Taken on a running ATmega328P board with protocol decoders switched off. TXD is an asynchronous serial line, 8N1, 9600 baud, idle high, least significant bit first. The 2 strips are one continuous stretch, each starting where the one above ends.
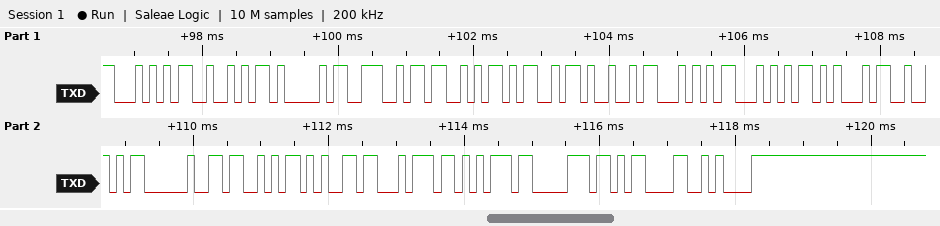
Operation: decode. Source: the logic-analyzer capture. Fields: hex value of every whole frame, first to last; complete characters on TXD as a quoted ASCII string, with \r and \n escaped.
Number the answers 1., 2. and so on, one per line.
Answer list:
1. 54 52 41 4E 53 4D 49 54 54 45 52 20 53 65 74 75 70 0D 0A
2. "TRANSMITTER Setup\r\n"
